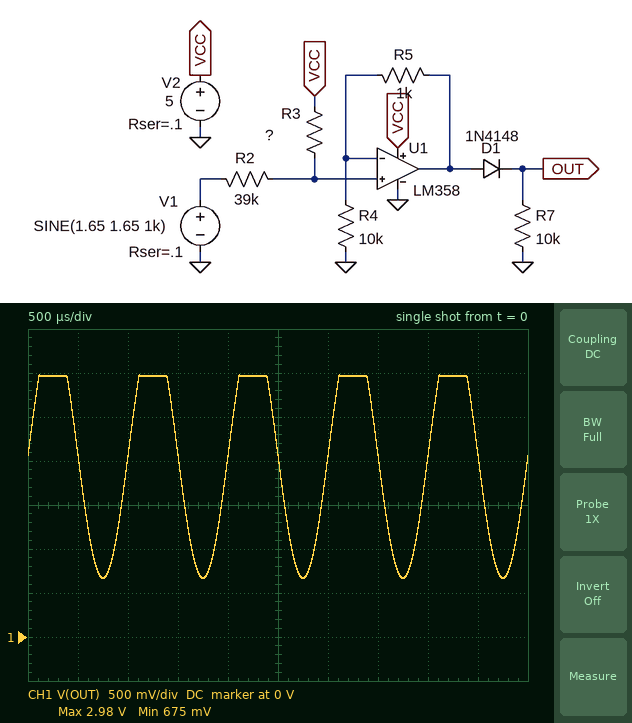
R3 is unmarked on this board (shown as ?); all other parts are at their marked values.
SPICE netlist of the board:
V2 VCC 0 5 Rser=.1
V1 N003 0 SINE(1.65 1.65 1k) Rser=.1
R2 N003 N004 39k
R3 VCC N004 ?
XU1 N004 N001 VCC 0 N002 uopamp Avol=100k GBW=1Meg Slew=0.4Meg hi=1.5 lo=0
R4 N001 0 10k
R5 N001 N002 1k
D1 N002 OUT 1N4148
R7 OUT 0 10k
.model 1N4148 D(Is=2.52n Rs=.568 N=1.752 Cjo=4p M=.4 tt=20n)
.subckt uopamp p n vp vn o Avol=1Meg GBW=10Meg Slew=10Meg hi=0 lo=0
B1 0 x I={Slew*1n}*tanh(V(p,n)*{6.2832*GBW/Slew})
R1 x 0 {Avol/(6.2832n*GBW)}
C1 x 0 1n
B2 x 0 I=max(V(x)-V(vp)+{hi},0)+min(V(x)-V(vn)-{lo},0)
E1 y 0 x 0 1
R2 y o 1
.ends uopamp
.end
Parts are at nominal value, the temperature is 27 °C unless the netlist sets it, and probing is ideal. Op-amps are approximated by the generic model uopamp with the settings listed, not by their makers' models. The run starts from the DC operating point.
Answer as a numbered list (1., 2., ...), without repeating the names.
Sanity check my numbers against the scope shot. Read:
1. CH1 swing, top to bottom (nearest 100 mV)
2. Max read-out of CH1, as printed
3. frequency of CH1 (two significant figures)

1. 2.3 V
2. 2.98 V
3. 1.0 kHz
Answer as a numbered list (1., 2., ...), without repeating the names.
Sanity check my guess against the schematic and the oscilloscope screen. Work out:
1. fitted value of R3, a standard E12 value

1. 150 kΩ
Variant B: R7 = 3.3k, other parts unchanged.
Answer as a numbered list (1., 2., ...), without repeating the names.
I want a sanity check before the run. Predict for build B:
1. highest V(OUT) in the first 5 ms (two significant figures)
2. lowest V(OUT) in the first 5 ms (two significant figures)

1. 2.9 V
2. 630 mV
